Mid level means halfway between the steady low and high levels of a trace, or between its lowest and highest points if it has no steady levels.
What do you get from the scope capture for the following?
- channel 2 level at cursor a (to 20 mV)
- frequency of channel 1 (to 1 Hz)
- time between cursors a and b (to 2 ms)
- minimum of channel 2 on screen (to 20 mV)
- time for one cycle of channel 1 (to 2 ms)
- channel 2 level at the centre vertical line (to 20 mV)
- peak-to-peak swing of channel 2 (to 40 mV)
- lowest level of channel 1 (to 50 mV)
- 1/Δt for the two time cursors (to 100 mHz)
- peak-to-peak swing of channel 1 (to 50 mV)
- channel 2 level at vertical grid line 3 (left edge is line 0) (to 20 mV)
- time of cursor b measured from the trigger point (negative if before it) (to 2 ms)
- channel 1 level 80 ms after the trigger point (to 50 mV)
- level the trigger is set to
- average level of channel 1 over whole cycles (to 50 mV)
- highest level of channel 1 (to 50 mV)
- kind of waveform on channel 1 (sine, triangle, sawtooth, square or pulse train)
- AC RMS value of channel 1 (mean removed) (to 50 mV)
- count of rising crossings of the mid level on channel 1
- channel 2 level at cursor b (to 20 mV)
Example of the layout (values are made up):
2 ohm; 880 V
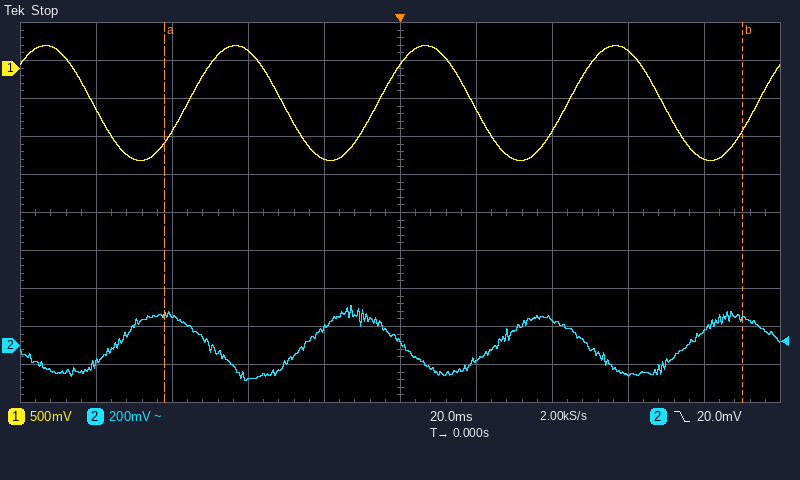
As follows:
160 mV; 20 Hz; 152 ms; -180 mV; 50 ms; 20 mV; 400 mV; -1.20 V; 6.6 Hz; 1.50 V; -180 mV; +90 ms; -1.20 V; 20.0 mV; -450 mV; 300 mV; sine; 550 mV; 4; 140 mV
